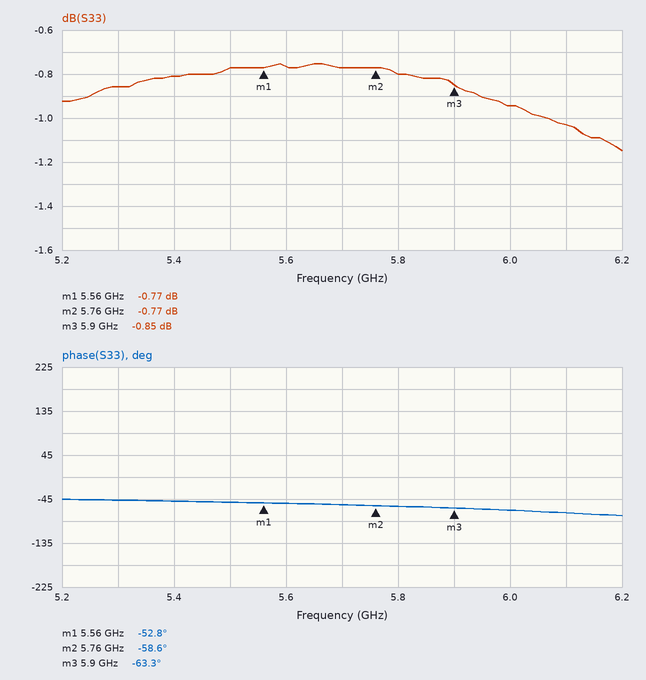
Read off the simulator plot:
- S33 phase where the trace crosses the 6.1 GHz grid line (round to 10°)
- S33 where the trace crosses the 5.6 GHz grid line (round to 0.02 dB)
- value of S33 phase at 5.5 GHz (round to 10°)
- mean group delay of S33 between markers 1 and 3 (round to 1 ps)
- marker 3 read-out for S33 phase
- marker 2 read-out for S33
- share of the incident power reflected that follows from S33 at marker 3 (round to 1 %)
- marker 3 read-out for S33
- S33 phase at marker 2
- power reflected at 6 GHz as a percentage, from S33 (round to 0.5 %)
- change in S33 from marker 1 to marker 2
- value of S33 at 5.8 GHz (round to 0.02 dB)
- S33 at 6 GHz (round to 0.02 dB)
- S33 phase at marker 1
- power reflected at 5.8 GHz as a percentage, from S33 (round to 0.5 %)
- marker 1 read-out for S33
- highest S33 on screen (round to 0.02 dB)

-70°
-0.76 dB
-50°
86 ps
-63.3°
-0.77 dB
82 %
-0.85 dB
-58.6°
80.5 %
0.00 dB
-0.80 dB
-0.94 dB
-52.8°
83.0 %
-0.77 dB
-0.76 dB
